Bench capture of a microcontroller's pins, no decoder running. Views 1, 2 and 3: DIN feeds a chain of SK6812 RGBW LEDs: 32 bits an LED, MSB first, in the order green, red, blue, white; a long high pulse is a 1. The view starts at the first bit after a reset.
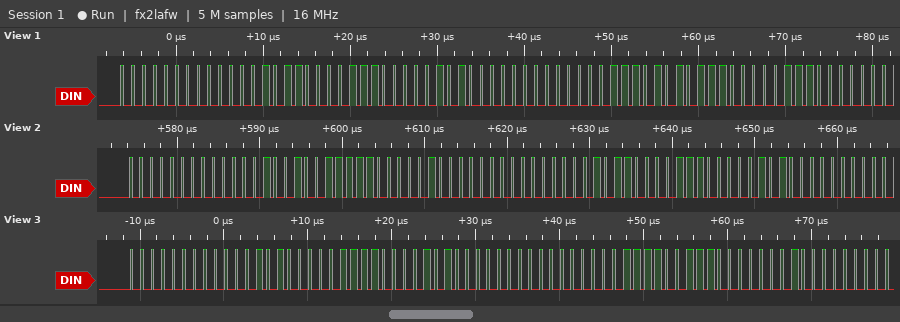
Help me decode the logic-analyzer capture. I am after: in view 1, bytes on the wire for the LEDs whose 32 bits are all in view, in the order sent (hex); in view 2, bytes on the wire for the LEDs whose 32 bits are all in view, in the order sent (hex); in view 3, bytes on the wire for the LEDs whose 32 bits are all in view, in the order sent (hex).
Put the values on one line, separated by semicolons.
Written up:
00 05 87 05 00 07 57 07; 00 04 9F 04 00 05 87 05; 00 0A 0F 0A 00 01 E7 01
